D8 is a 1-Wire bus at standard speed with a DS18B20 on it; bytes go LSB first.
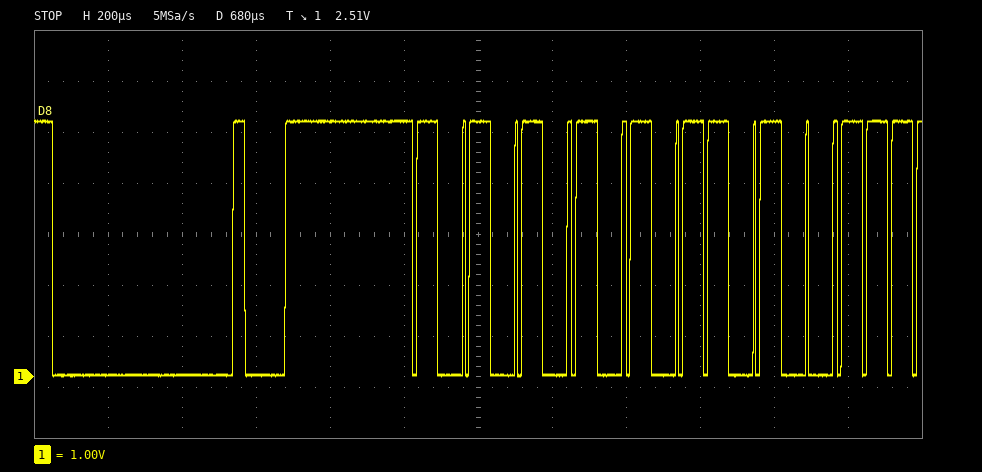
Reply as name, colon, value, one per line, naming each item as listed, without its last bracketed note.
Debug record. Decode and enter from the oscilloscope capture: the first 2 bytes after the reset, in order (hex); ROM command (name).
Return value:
the first 2 bytes after the reset, in order: 55 2D
ROM command: Match ROM
